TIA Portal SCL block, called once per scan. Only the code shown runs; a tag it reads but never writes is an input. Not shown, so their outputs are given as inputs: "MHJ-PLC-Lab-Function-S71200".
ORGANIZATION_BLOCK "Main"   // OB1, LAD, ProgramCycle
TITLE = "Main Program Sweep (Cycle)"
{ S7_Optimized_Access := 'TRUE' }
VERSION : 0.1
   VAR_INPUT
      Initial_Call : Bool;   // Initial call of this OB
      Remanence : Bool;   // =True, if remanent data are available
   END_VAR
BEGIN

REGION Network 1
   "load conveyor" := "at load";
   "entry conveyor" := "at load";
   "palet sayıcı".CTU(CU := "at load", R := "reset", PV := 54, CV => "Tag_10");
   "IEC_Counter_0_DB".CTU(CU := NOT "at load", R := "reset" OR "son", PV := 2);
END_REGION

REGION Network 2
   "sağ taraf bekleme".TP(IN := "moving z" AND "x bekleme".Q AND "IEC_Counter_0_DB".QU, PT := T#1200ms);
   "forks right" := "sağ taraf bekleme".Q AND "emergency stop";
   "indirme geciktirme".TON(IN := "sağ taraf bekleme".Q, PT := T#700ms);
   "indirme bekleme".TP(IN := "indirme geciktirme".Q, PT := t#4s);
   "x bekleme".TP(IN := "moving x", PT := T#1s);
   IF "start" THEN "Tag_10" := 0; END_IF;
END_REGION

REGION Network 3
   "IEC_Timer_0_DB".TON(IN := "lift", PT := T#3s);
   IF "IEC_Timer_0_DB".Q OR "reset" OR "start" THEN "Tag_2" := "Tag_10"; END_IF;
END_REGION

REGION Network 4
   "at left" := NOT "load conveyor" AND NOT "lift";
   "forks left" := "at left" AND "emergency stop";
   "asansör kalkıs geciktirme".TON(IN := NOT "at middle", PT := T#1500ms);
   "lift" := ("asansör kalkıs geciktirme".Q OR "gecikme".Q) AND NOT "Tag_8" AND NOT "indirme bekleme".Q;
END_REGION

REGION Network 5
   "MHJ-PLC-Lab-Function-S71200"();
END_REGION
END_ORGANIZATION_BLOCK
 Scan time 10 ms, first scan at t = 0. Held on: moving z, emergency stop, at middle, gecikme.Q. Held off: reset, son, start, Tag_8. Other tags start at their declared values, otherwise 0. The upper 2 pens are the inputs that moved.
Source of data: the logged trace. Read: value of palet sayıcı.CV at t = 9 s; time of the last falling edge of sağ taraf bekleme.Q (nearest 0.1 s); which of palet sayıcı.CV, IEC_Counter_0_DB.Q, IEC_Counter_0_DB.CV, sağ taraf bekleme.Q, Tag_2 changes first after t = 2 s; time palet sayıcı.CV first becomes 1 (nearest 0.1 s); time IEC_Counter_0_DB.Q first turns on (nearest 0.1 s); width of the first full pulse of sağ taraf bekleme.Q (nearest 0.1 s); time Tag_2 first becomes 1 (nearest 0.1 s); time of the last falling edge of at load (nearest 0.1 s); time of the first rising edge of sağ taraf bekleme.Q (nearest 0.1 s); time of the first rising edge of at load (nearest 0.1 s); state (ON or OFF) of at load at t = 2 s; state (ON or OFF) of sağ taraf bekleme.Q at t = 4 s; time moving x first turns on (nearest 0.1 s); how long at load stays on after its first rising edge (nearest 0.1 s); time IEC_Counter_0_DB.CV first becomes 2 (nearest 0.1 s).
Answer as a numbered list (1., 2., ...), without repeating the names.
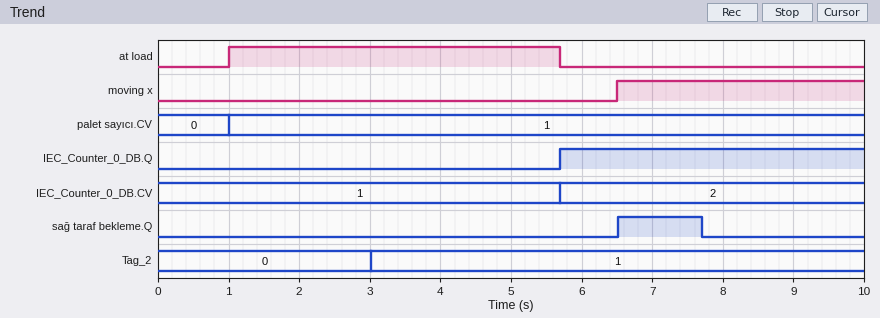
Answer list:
1. 1
2. 7.7 s
3. Tag_2
4. 1.0 s
5. 5.7 s
6. 1.2 s
7. 3.0 s
8. 5.7 s
9. 6.5 s
10. 1.0 s
11. ON
12. OFF
13. 6.5 s
14. 4.7 s
15. 5.7 s
